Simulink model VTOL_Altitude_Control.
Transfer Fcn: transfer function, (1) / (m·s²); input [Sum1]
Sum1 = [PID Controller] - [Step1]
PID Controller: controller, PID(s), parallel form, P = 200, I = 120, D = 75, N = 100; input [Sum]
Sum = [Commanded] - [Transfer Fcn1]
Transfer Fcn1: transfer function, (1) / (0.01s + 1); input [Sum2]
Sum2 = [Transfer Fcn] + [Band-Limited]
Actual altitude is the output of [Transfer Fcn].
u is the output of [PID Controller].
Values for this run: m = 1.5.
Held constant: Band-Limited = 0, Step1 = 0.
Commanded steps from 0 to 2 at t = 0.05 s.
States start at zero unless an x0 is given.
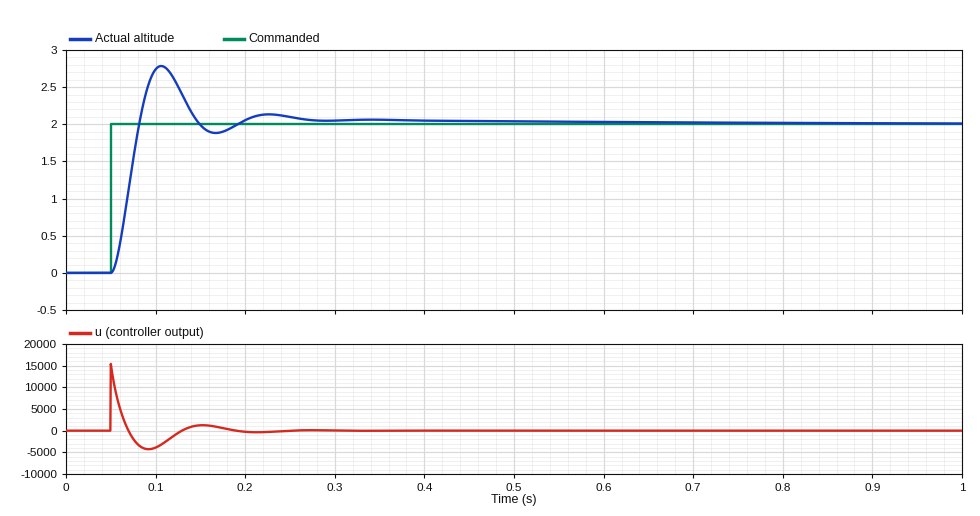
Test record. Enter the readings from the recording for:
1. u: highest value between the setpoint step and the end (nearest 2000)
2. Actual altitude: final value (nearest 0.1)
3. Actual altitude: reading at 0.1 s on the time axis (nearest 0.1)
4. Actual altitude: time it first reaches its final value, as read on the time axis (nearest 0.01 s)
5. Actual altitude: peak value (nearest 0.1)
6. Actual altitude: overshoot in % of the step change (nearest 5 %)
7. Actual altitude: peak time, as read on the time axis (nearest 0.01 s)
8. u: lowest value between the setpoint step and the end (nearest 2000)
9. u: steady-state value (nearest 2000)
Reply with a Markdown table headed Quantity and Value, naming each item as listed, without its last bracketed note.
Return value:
| Quantity | Value |
|---|---|
| u: highest value between the setpoint step and the end | 16000 |
| Actual altitude: final value | 2.0 |
| Actual altitude: reading at 0.1 s on the time axis | 2.7 |
| Actual altitude: time it first reaches its final value, as read on the time axis | 0.08 s |
| Actual altitude: peak value | 2.8 |
| Actual altitude: overshoot in % of the step change | 40 % |
| Actual altitude: peak time, as read on the time axis | 0.11 s |
| u: lowest value between the setpoint step and the end | -4000 |
| u: steady-state value | 0 |
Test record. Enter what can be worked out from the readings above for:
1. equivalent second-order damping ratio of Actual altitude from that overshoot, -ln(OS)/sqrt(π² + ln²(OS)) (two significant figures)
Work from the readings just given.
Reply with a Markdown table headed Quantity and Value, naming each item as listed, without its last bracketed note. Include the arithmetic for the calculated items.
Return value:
| Quantity | Value |
|---|---|
| equivalent second-order damping ratio of Actual altitude from that overshoot, -ln(OS)/sqrt(π² + ln²(OS)) | ln(0.4) = -0.916; 0.916 / sqrt(9.870 + 0.840) = 0.28 |
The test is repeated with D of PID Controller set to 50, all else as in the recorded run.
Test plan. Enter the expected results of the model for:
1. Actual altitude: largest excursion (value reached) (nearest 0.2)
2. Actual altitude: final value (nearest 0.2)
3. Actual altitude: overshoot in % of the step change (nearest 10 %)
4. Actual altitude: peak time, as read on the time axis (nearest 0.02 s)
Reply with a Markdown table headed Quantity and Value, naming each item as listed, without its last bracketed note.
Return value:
| Quantity | Value |
|---|---|
| Actual altitude: largest excursion (value reached) | 2.6 |
| Actual altitude: final value | 2.0 |
| Actual altitude: overshoot in % of the step change | 30 % |
| Actual altitude: peak time, as read on the time axis | 0.12 s |
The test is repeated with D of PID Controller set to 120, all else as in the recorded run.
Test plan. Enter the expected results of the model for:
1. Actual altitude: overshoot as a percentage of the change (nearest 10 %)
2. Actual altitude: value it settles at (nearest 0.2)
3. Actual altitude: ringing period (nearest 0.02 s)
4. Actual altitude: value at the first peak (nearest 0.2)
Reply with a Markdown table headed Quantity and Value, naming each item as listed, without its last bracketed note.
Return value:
| Quantity | Value |
|---|---|
| Actual altitude: overshoot as a percentage of the change | 60 % |
| Actual altitude: value it settles at | 2.0 |
| Actual altitude: ringing period | 0.10 s |
| Actual altitude: value at the first peak | 3.2 |
